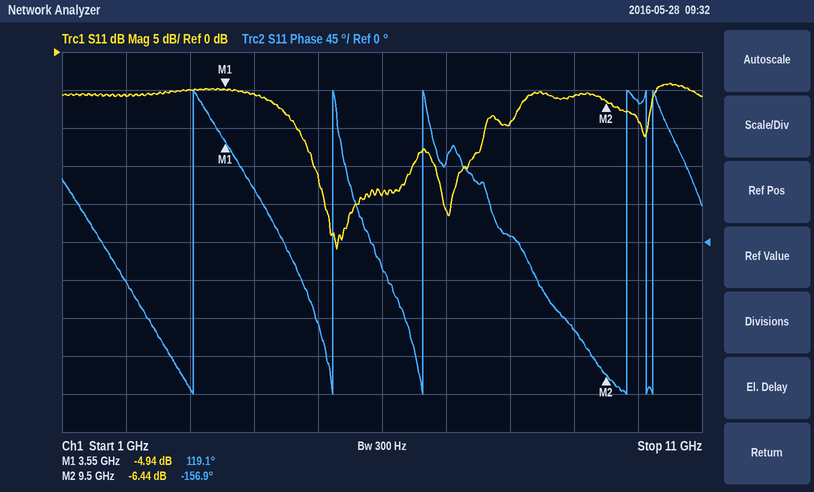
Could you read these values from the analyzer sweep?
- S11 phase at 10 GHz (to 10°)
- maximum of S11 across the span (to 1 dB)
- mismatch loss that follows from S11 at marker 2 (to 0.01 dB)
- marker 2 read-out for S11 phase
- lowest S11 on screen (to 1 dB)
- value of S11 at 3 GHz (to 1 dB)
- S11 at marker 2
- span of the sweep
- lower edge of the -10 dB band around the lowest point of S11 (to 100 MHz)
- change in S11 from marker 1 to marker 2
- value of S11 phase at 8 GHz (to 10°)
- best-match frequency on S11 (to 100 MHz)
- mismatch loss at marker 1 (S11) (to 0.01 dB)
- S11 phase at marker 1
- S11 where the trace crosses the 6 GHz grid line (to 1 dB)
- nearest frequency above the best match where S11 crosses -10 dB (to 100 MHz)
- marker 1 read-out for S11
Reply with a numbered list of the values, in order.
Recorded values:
1. 170°
2. -4 dB
3. 1.12 dB
4. -156.9°
5. -26 dB
6. -5 dB
7. -6.44 dB
8. 10 GHz
9. 4.7 GHz
10. -1.50 dB
11. 10°
12. 5.3 GHz
13. 1.68 dB
14. 119.1°
15. -19 dB
16. 7.6 GHz
17. -4.94 dB
